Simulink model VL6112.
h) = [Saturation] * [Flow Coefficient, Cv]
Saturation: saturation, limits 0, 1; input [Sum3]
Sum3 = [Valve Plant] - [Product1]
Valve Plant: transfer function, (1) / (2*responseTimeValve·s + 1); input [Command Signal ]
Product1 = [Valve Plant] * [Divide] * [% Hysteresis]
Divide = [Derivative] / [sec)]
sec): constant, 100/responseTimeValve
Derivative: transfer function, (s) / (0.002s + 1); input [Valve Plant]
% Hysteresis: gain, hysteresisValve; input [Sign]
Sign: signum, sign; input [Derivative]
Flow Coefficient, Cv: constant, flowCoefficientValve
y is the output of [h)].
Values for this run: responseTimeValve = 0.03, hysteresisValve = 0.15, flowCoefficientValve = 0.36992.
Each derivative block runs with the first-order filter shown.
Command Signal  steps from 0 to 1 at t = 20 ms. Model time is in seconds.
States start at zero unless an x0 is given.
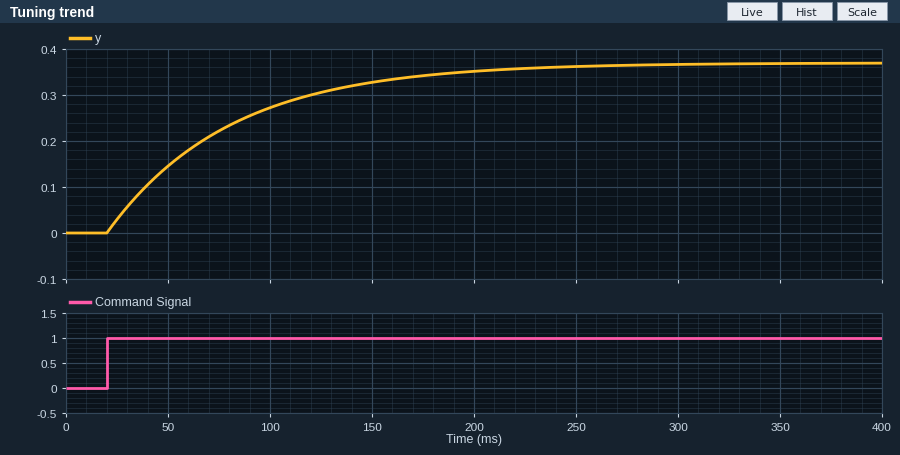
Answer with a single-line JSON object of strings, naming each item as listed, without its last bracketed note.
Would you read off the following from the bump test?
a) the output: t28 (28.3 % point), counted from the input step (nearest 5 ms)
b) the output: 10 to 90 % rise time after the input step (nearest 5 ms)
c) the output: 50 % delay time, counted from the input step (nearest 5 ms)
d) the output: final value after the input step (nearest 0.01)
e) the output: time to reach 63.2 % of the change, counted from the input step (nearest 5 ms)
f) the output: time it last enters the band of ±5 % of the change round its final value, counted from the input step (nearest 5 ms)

{"the output: t28 (28.3 % point), counted from the input step": "20 ms", "the output: 10 to 90 % rise time after the input step": "130 ms", "the output: 50 % delay time, counted from the input step": "40 ms", "the output: final value after the input step": "0.37", "the output: time to reach 63.2 % of the change, counted from the input step": "60 ms", "the output: time it last enters the band of ±5 % of the change round its final value, counted from the input step": "180 ms"}
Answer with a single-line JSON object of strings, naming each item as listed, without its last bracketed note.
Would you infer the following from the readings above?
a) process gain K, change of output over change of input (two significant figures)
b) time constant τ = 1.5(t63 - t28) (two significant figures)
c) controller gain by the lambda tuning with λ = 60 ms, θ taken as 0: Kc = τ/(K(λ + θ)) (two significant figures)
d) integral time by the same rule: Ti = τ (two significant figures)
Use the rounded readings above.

{"process gain K, change of output over change of input": "0.37", "time constant τ = 1.5(t63 - t28)": "60 ms", "controller gain by the lambda tuning with λ = 60 ms, θ taken as 0: Kc = τ/(K(λ + θ))": "2.7", "integral time by the same rule: Ti = τ": "60 ms"}
